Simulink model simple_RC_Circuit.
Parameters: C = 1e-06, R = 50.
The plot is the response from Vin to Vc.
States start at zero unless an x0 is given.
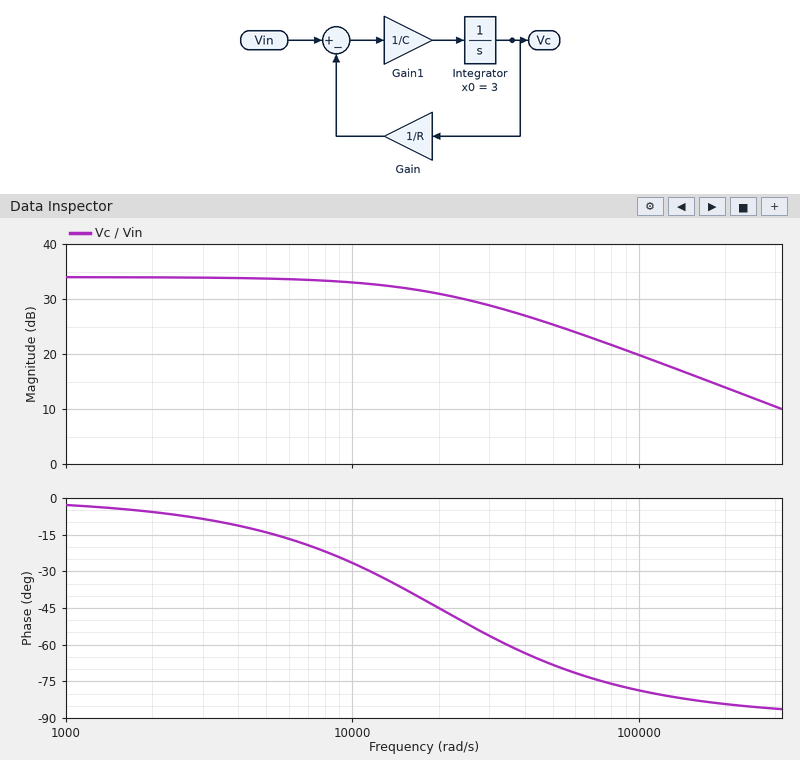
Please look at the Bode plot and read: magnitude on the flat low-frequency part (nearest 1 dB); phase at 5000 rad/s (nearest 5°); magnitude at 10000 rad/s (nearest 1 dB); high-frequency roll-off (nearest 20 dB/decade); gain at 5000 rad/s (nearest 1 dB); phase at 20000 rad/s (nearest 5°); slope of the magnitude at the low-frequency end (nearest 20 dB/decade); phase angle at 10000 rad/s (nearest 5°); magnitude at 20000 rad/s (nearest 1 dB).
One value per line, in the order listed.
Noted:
34 dB
-15°
33 dB
-20 dB/decade
34 dB
-45°
0 dB/decade
-25°
31 dB
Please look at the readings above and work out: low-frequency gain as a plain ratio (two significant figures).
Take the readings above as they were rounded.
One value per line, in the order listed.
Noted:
50
